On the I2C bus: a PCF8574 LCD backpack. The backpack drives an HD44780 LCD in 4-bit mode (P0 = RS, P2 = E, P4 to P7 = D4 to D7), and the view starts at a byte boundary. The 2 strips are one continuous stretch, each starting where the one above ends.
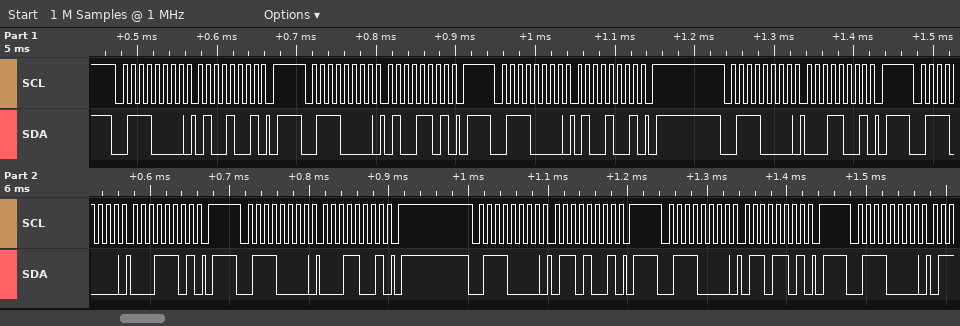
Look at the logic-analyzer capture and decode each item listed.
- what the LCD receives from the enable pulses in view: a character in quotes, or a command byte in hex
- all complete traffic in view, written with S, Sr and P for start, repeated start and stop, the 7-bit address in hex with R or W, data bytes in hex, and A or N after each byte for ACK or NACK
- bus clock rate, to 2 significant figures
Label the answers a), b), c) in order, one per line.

a) 'A'
b) S 38W A 49 A P S 38W A 4D A P S 38W A 49 A P S 38W A 19 A P S 38W A 1D A P S 38W A 19 A P S 38W A 69 A P S 38W A 6D A P S 38W A
c) 100 kHz
